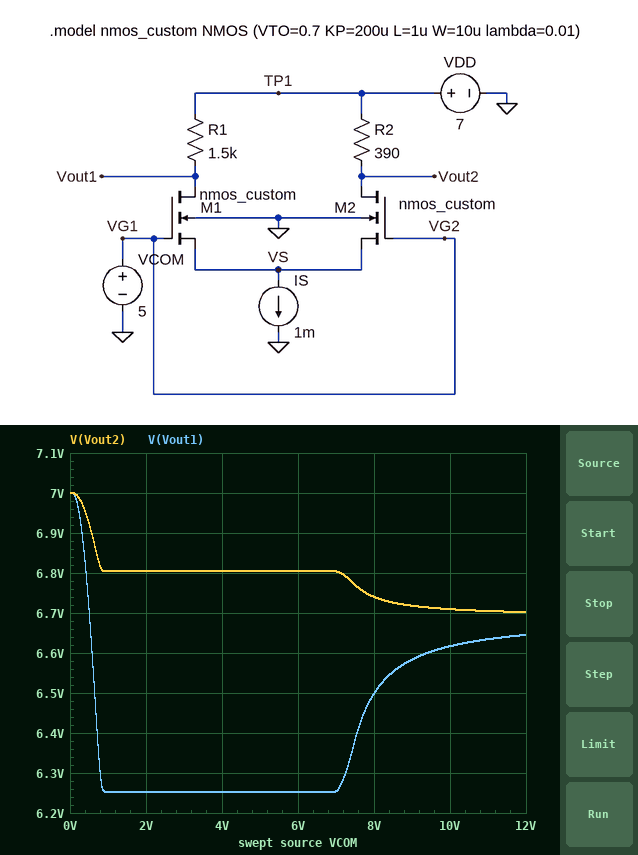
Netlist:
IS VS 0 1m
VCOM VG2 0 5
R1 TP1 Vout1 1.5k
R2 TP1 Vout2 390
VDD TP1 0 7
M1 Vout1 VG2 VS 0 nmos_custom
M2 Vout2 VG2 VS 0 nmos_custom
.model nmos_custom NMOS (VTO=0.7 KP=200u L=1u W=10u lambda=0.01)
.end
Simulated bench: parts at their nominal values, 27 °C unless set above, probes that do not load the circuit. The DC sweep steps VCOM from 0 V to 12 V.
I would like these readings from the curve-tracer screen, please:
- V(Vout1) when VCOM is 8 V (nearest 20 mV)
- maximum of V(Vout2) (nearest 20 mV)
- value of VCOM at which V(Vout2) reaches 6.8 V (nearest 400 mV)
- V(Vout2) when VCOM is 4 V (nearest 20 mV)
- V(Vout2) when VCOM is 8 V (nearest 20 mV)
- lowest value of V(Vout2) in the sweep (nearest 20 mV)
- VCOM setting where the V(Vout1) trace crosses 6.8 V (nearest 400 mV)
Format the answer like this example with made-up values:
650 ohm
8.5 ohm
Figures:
6.50 V
7.00 V
7.2 V
6.80 V
6.74 V
6.70 V
400 mV
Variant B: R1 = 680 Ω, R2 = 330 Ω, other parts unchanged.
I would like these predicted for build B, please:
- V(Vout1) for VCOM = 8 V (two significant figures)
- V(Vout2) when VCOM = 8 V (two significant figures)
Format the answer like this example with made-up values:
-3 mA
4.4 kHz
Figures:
6.7 V
6.8 V
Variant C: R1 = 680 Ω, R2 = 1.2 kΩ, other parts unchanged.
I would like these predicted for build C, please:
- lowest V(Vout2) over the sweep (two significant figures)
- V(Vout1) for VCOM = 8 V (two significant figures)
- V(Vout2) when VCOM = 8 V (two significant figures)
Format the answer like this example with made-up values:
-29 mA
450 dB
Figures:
6.4 V
6.6 V
6.5 V
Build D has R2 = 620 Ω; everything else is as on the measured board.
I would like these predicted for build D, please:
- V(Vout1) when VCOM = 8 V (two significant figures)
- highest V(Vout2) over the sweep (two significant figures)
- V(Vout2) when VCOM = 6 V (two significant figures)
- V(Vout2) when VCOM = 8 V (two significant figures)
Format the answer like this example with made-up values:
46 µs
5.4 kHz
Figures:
6.4 V
7.0 V
6.7 V
6.6 V
